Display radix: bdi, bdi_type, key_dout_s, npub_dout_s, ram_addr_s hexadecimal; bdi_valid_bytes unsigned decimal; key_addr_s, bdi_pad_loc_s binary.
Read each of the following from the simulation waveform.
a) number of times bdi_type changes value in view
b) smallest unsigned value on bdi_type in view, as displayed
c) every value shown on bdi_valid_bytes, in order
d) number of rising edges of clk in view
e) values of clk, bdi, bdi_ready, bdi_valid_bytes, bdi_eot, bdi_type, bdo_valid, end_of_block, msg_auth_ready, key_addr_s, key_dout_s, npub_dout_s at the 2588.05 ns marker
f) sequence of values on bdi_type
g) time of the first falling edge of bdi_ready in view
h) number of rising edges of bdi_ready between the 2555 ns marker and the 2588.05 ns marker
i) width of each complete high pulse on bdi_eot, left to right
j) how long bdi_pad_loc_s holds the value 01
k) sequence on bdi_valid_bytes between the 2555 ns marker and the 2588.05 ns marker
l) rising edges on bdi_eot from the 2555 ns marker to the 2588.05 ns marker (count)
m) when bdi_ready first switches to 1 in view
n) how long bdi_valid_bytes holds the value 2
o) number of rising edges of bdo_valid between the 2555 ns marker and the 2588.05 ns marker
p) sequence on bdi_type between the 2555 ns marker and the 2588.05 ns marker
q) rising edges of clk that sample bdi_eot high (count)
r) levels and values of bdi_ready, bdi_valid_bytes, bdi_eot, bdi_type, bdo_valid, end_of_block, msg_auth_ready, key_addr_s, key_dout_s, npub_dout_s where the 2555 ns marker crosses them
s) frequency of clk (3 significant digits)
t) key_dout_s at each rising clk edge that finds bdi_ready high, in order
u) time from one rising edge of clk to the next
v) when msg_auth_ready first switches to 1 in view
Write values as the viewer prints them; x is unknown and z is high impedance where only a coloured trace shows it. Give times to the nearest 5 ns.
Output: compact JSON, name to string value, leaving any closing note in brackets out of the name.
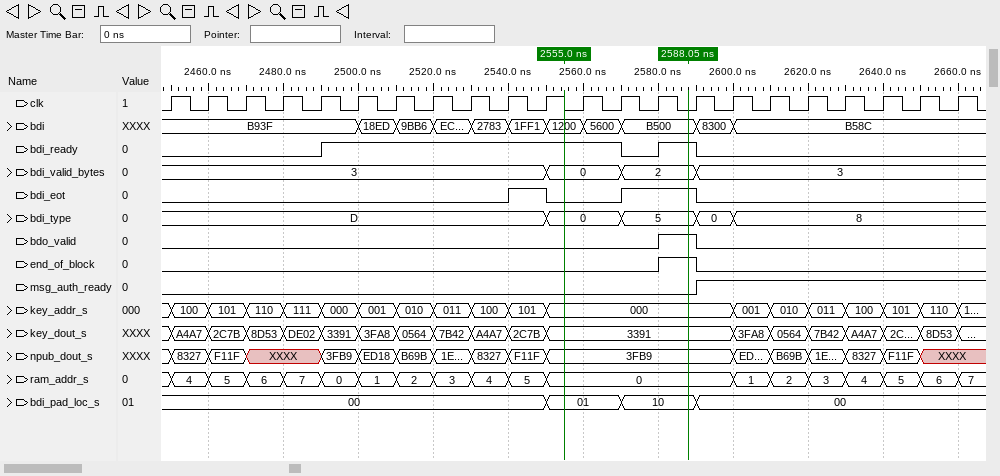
{"number of times bdi_type changes value in view": "4", "smallest unsigned value on bdi_type in view, as displayed": "0", "every value shown on bdi_valid_bytes, in order": "3, 0, 2, 3", "number of rising edges of clk in view": "22", "values of clk, bdi, bdi_ready, bdi_valid_bytes, bdi_eot, bdi_type, bdo_valid, end_of_block, msg_auth_ready, key_addr_s, key_dout_s, npub_dout_s at the 2588.05 ns marker": "clk=0, bdi=B500, bdi_ready=1, bdi_valid_bytes=2, bdi_eot=1, bdi_type=5, bdo_valid=1, end_of_block=1, msg_auth_ready=0, key_addr_s=000, key_dout_s=3391, npub_dout_s=3FB9", "sequence of values on bdi_type": "D, 0, 5, 0, 8", "time of the first falling edge of bdi_ready in view": "2570 ns", "number of rising edges of bdi_ready between the 2555 ns marker and the 2588.05 ns marker": "1", "width of each complete high pulse on bdi_eot, left to right": "10 ns, 20 ns", "how long bdi_pad_loc_s holds the value 01": "20 ns", "sequence on bdi_valid_bytes between the 2555 ns marker and the 2588.05 ns marker": "0, 2", "rising edges on bdi_eot from the 2555 ns marker to the 2588.05 ns marker": "1", "when bdi_ready first switches to 1 in view": "2490 ns", "how long bdi_valid_bytes holds the value 2": "20 ns", "number of rising edges of bdo_valid between the 2555 ns marker and the 2588.05 ns marker": "1", "sequence on bdi_type between the 2555 ns marker and the 2588.05 ns marker": "0, 5", "rising edges of clk that sample bdi_eot high": "3", "levels and values of bdi_ready, bdi_valid_bytes, bdi_eot, bdi_type, bdo_valid, end_of_block, msg_auth_ready, key_addr_s, key_dout_s, npub_dout_s where the 2555 ns marker crosses them": "bdi_ready=1, bdi_valid_bytes=0, bdi_eot=0, bdi_type=0, bdo_valid=0, end_of_block=0, msg_auth_ready=0, key_addr_s=000, key_dout_s=3391, npub_dout_s=3FB9", "frequency of clk": "100 MHz", "key_dout_s at each rising clk edge that finds bdi_ready high, in order": "3391, 3FA8, 0564, 7B42, A4A7, 2C7B, 3391, 3391, 3391", "time from one rising edge of clk to the next": "10 ns", "when msg_auth_ready first switches to 1 in view": "2590 ns"}
